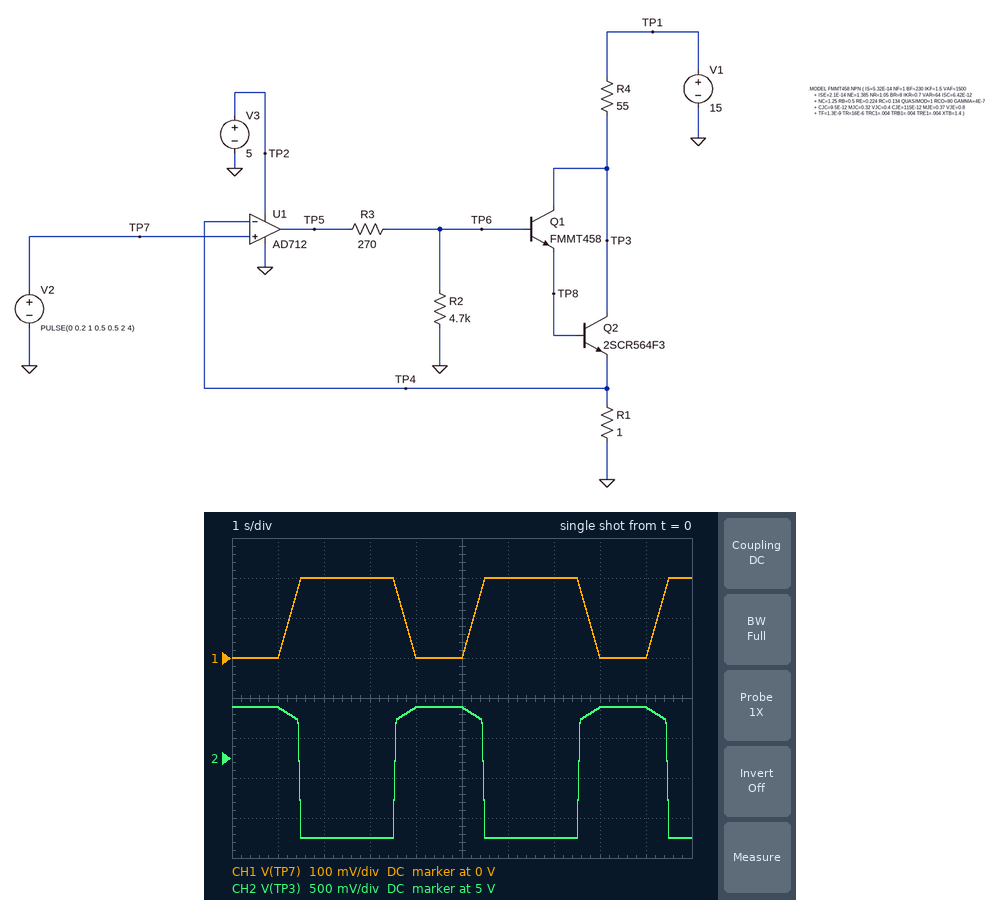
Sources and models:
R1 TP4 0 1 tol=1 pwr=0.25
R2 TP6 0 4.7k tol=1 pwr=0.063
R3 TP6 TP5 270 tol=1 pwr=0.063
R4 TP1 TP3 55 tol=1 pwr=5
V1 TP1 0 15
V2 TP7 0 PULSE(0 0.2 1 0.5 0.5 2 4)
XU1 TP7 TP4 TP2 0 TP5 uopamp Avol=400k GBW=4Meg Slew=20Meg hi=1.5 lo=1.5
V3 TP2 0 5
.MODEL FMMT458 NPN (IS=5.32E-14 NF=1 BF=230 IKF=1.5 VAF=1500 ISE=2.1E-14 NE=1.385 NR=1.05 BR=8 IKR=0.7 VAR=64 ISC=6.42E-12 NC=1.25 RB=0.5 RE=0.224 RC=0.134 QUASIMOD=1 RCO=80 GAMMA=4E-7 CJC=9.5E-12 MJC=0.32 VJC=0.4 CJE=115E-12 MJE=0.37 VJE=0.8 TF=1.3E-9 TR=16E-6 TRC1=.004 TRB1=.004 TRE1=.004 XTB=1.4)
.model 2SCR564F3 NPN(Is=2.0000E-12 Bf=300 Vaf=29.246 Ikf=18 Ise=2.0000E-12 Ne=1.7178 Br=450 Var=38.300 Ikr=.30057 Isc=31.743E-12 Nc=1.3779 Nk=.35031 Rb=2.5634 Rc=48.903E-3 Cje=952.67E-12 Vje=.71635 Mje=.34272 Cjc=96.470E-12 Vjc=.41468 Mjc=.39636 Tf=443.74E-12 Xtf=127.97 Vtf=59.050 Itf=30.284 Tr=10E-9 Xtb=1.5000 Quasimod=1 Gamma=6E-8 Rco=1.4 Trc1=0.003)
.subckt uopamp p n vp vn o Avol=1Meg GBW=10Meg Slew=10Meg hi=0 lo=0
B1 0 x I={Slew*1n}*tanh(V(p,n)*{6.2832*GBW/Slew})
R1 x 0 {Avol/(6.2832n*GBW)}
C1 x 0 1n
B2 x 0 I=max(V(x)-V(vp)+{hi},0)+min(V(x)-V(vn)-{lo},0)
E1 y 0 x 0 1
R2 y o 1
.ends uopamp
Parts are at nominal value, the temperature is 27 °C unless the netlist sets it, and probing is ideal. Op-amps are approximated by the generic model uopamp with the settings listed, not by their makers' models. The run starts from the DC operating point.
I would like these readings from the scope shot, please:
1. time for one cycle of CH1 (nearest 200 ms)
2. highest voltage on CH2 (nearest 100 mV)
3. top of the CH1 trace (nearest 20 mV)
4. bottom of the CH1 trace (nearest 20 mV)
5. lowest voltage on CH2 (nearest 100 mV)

4.0 s
5.6 V
200 mV
0 V
4.0 V
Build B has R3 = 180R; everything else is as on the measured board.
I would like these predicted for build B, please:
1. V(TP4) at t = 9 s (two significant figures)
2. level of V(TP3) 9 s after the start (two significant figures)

190 mV
4.6 V
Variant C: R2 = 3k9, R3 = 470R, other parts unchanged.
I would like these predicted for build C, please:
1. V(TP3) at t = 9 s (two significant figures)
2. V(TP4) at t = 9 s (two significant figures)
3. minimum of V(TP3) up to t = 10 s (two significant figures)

8.6 V
120 mV
4.0 V
